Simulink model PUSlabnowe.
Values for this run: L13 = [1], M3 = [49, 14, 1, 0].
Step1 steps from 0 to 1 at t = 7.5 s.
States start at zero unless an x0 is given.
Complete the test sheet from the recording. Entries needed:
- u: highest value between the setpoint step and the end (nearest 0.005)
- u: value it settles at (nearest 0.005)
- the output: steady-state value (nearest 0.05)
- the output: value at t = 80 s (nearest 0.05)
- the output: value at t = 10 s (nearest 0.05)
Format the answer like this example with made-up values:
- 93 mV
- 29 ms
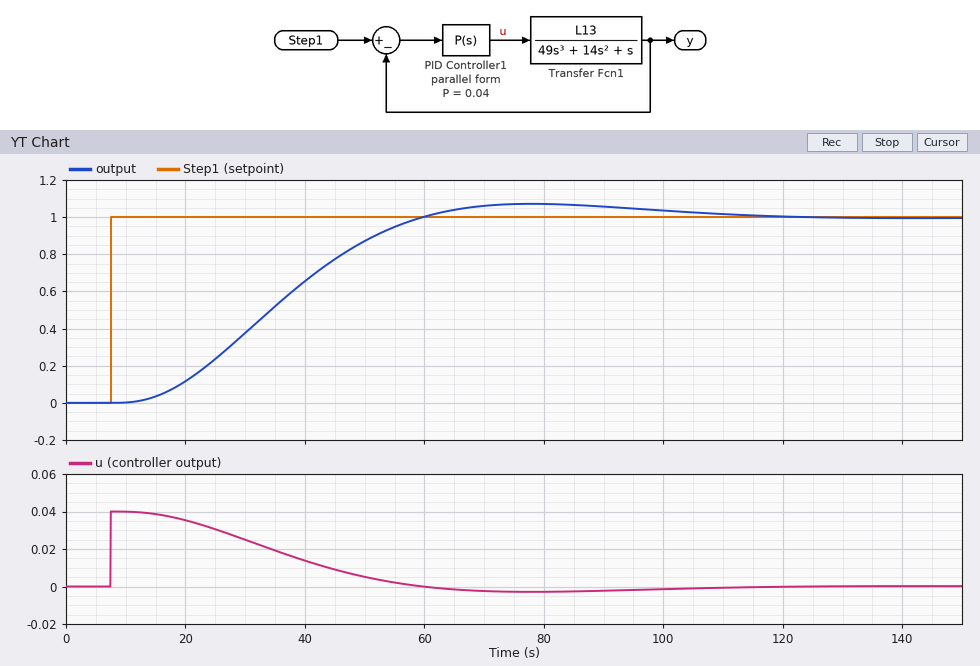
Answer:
- 0.040
- 0.000
- 1.00
- 1.05
- 0.00
